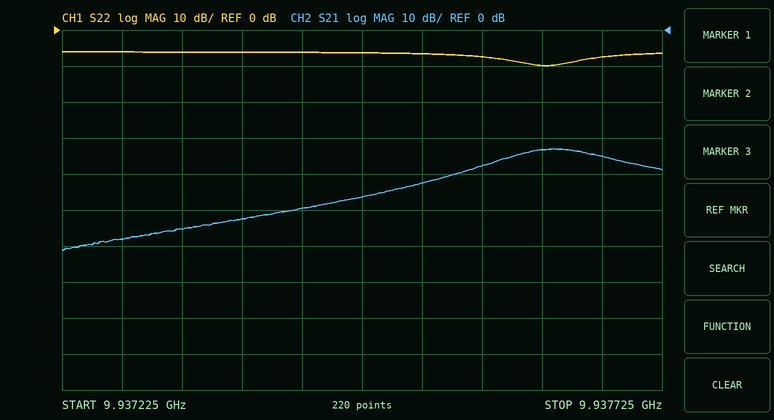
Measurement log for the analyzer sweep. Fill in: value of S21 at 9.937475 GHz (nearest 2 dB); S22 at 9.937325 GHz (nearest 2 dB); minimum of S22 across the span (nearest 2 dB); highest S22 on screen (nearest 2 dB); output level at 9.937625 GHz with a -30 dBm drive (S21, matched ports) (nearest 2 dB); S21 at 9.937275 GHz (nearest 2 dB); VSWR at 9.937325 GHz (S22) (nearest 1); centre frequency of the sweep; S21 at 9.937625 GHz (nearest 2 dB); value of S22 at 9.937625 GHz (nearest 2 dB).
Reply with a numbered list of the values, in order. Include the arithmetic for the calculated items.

1. -46 dB
2. -6 dB
3. -10 dB
4. -6 dB
5. -30 dBm + (-34 dB) = -64 dBm
6. -58 dB
7. |Γ| = 10^(-6/20) = 0.5012; VSWR = (1 + 0.5012)/(1 − 0.5012) ≈ 3
8. 9.937475 GHz
9. -34 dB
10. -10 dB
